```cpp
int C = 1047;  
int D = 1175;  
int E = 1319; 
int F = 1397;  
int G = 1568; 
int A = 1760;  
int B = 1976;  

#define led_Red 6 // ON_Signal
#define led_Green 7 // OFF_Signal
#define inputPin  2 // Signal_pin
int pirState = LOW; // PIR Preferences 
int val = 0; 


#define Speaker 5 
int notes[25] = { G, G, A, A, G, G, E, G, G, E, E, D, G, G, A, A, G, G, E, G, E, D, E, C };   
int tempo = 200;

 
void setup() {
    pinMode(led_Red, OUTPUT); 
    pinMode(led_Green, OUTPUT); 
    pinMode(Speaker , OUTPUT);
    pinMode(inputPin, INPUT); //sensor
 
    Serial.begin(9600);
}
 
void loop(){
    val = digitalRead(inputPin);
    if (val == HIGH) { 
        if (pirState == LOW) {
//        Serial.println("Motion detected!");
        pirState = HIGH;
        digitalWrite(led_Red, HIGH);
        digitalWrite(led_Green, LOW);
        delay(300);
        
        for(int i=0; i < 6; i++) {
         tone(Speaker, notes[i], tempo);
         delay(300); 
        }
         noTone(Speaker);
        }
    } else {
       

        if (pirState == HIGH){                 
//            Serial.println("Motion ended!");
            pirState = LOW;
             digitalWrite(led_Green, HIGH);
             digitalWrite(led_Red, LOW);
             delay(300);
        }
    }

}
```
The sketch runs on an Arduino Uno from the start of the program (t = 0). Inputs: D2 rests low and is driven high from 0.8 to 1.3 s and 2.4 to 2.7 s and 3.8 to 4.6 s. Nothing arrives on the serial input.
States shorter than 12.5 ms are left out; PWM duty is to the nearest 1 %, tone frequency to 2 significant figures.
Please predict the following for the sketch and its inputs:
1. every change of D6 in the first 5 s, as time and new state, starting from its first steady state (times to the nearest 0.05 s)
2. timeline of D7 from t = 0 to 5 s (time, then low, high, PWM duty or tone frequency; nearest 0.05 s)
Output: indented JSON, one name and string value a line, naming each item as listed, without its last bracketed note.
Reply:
{
  "every change of D6 in the first 5 s, as time and new state, starting from its first steady state": "0 s low; 0.8 s high; 2.9 s low; 3.8 s high",
  "timeline of D7 from t = 0 to 5 s": "0 s low; 2.9 s high; 3.8 s low"
}
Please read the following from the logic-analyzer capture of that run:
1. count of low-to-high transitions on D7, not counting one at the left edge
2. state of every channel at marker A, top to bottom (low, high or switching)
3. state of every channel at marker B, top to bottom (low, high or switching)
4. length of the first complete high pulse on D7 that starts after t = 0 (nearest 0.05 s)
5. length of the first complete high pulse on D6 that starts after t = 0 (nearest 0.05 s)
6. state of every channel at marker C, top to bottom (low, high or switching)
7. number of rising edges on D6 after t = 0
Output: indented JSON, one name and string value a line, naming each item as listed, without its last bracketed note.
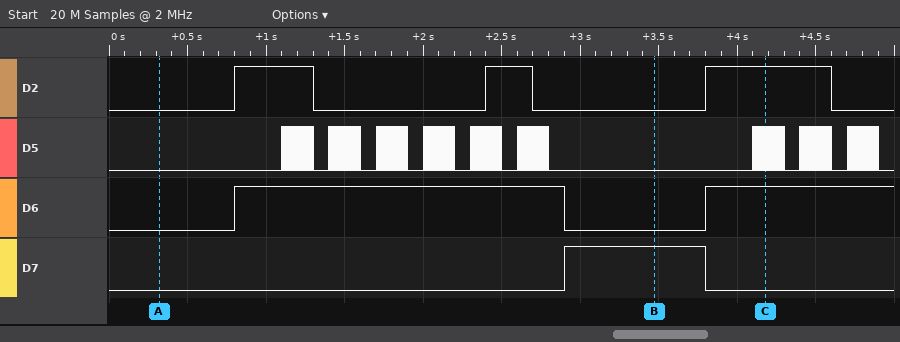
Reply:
{
  "count of low-to-high transitions on D7, not counting one at the left edge": "1",
  "state of every channel at marker A, top to bottom": "D2 low, D5 low, D6 low, D7 low",
  "state of every channel at marker B, top to bottom": "D2 low, D5 low, D6 low, D7 high",
  "length of the first complete high pulse on D7 that starts after t = 0": "0.90 s",
  "length of the first complete high pulse on D6 that starts after t = 0": "2.10 s",
  "state of every channel at marker C, top to bottom": "D2 high, D5 switching, D6 high, D7 low",
  "number of rising edges on D6 after t = 0": "2"
}
